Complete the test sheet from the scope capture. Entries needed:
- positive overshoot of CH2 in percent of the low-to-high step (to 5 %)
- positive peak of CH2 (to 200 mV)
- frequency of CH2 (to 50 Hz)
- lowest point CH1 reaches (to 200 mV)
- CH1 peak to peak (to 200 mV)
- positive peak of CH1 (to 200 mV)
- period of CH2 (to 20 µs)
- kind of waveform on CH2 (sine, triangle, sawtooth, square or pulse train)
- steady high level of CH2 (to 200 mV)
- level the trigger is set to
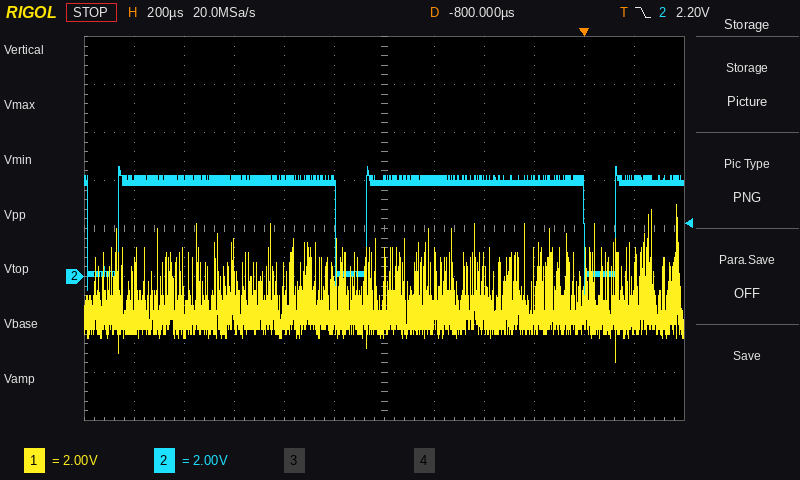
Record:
15 %
4.6 V
1.00 kHz
-3.6 V
6.6 V
3.0 V
1.00 ms
pulse train
4.0 V
2.20 V
